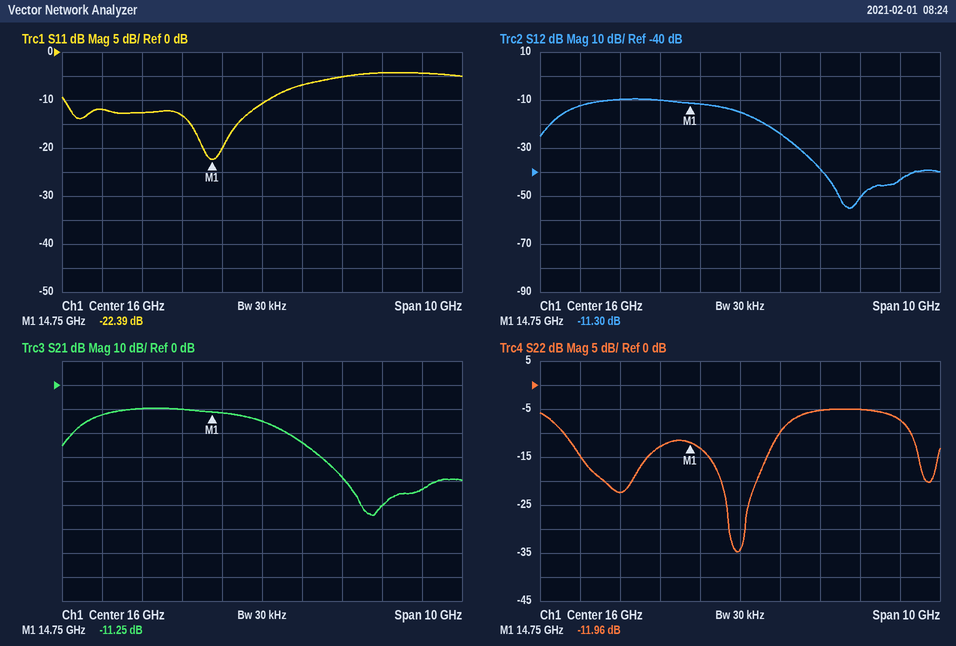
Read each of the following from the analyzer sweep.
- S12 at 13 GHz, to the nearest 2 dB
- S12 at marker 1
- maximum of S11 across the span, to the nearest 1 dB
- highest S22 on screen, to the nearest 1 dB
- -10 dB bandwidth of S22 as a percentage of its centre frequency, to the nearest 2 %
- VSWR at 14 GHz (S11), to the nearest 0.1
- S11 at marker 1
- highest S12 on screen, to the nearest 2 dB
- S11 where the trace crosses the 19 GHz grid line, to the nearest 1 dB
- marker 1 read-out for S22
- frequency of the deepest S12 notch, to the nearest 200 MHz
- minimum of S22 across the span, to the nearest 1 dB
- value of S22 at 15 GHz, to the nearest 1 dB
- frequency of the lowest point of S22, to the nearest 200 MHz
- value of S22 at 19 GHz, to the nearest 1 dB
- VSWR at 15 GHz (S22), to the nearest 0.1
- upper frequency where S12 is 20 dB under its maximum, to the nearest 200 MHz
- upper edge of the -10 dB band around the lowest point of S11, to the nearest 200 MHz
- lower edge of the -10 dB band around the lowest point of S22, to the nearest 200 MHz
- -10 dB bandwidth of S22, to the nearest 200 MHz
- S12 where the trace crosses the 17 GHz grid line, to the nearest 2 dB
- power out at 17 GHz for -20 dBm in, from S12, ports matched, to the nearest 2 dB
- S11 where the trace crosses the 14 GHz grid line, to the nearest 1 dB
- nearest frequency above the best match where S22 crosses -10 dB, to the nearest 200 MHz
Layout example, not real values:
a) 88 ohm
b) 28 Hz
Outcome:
a) -10 dB
b) -11.30 dB
c) -4 dB
d) -5 dB
e) 38 %
f) 1.6
g) -22.39 dB
h) -10 dB
i) -4 dB
j) -11.96 dB
k) 18.8 GHz
l) -35 dB
m) -13 dB
n) 16.0 GHz
o) -5 dB
p) 1.6
q) 17.4 GHz
r) 16.2 GHz
s) 11.6 GHz
t) 5.4 GHz
u) -24 dB
v) -44 dBm
w) -13 dB
x) 17.0 GHz
